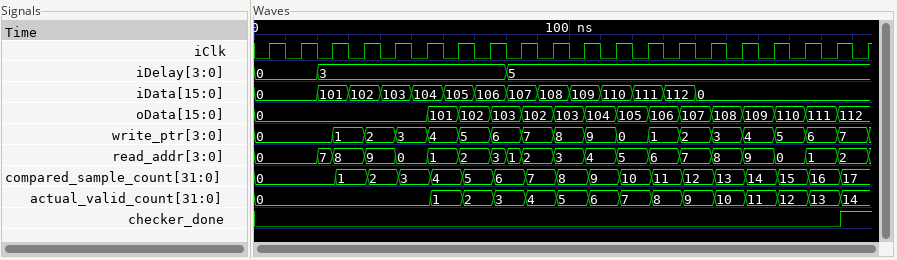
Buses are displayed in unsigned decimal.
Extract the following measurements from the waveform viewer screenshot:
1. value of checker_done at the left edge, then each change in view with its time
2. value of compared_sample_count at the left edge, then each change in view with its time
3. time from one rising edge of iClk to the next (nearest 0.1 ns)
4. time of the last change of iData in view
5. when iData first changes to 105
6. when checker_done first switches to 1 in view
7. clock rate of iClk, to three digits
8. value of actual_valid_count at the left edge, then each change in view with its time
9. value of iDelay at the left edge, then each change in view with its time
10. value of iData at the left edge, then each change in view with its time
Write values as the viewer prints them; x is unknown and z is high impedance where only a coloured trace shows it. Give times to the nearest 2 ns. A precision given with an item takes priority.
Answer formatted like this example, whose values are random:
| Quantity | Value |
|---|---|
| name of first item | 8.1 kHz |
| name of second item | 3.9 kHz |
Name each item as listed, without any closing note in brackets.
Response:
| Quantity | Value |
|---|---|
| value of checker_done at the left edge, then each change in view with its time | 0, 1 at 186 ns |
| value of compared_sample_count at the left edge, then each change in view with its time | 0, 1 at 26 ns, 2 at 36 ns, 3 at 46 ns, 4 at 56 ns, 5 at 66 ns, 6 at 76 ns, 7 at 86 ns, 8 at 96 ns, 9 at 106 ns, 10 at 116 ns, 11 at 126 ns, 12 at 136 ns, 13 at 146 ns, 14 at 156 ns, 15 at 166 ns, 16 at 176 ns, 17 at 186 ns |
| time from one rising edge of iClk to the next | 10 ns |
| time of the last change of iData in view | 140 ns |
| when iData first changes to 105 | 60 ns |
| when checker_done first switches to 1 in view | 186 ns |
| clock rate of iClk, to three digits | 100 MHz |
| value of actual_valid_count at the left edge, then each change in view with its time | 0, 1 at 56 ns, 2 at 66 ns, 3 at 76 ns, 4 at 86 ns, 5 at 96 ns, 6 at 106 ns, 7 at 116 ns, 8 at 126 ns, 9 at 136 ns, 10 at 146 ns, 11 at 156 ns, 12 at 166 ns, 13 at 176 ns, 14 at 186 ns |
| value of iDelay at the left edge, then each change in view with its time | 0, 3 at 20 ns, 5 at 80 ns |
| value of iData at the left edge, then each change in view with its time | 0, 101 at 20 ns, 102 at 30 ns, 103 at 40 ns, 104 at 50 ns, 105 at 60 ns, 106 at 70 ns, 107 at 80 ns, 108 at 90 ns, 109 at 100 ns, 110 at 110 ns, 111 at 120 ns, 112 at 130 ns, 0 at 140 ns |
